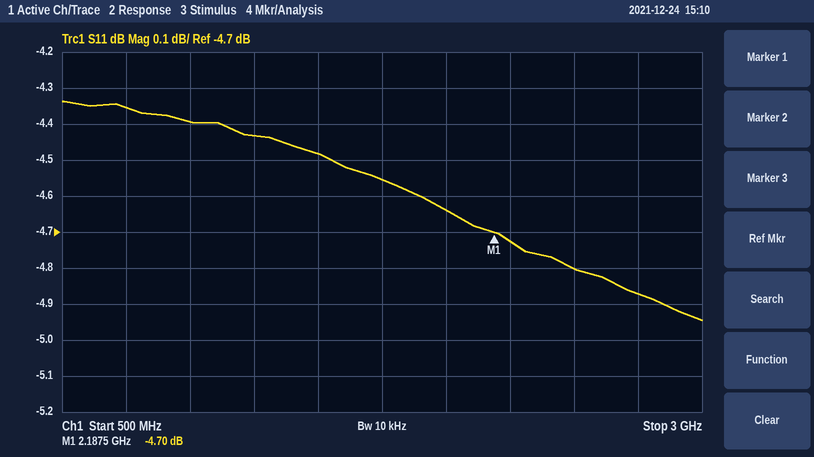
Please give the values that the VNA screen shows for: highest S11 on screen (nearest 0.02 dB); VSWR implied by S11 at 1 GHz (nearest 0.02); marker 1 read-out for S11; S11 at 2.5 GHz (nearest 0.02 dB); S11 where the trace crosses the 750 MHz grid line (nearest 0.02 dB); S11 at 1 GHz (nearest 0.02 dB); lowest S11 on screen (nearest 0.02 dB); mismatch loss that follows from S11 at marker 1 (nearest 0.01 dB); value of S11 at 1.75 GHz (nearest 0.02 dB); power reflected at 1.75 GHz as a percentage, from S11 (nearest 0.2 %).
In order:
-4.34 dB
4.04
-4.70 dB
-4.80 dB
-4.36 dB
-4.40 dB
-4.94 dB
1.80 dB
-4.56 dB
35.0 %
